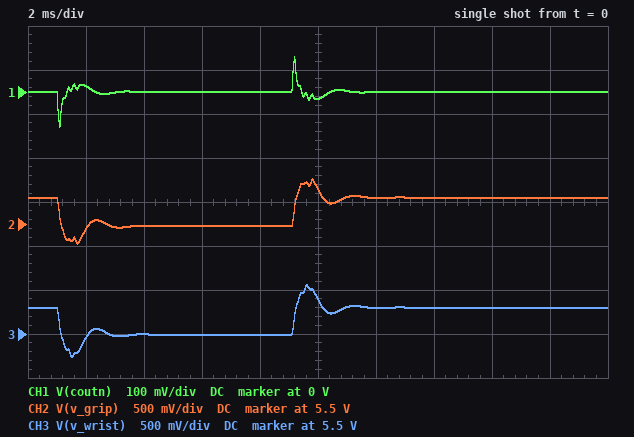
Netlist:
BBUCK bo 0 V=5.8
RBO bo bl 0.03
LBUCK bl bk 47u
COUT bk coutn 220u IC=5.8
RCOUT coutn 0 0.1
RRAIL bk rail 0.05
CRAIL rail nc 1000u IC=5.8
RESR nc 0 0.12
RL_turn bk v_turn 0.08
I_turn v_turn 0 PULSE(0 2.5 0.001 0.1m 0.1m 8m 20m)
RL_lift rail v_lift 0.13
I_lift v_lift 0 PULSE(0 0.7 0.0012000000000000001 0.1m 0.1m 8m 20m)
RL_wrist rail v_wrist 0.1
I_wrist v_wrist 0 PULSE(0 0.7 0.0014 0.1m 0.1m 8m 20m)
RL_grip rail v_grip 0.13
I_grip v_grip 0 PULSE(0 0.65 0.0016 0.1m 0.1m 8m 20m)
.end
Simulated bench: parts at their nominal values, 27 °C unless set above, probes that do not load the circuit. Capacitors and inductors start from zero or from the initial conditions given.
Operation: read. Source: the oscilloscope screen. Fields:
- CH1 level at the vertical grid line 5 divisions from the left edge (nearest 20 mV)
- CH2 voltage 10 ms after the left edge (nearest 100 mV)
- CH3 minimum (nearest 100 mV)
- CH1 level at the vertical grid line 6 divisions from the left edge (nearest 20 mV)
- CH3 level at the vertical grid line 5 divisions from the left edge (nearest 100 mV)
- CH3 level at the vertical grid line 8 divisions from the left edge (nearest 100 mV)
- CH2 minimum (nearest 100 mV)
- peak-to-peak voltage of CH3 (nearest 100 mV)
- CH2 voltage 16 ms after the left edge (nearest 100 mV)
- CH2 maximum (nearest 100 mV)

-20 mV
5.9 V
5.2 V
0 V
5.9 V
5.8 V
5.3 V
800 mV
5.8 V
6.0 V
